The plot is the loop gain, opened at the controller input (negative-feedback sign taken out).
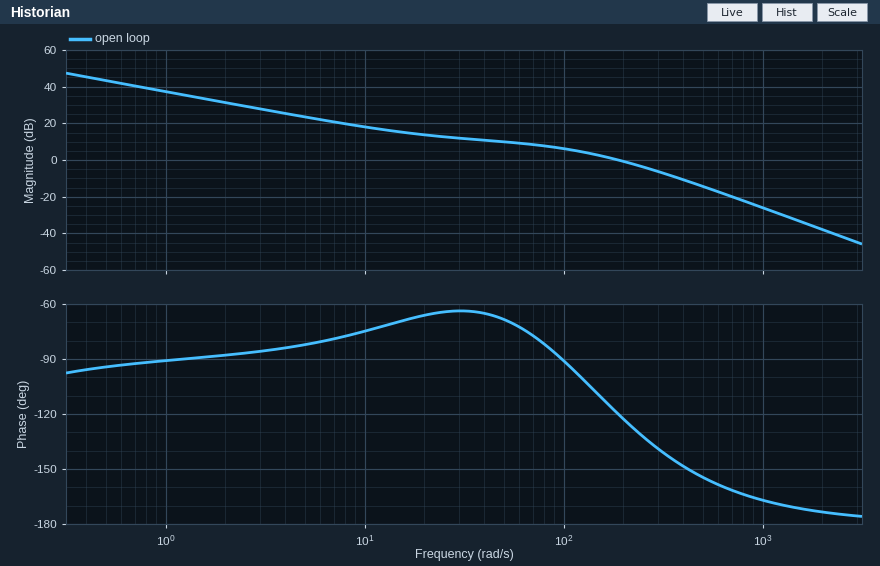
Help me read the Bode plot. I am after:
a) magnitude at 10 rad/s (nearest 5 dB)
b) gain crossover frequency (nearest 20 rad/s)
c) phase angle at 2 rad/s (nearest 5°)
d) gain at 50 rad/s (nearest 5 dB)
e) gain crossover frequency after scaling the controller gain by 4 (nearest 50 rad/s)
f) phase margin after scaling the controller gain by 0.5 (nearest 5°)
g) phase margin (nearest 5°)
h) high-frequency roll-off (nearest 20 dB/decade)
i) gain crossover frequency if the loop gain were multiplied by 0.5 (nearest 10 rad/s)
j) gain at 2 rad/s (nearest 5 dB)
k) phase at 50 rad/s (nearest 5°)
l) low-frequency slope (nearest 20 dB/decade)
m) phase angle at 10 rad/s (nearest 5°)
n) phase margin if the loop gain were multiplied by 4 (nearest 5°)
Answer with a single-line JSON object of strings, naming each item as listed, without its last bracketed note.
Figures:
{"magnitude at 10 rad/s": "20 dB", "gain crossover frequency": "180 rad/s", "phase angle at 2 rad/s": "-90°", "gain at 50 rad/s": "10 dB", "gain crossover frequency after scaling the controller gain by 4": "450 rad/s", "phase margin after scaling the controller gain by 0.5": "90°", "phase margin": "60°", "high-frequency roll-off": "-40 dB/decade", "gain crossover frequency if the loop gain were multiplied by 0.5": "100 rad/s", "gain at 2 rad/s": "30 dB", "phase at 50 rad/s": "-70°", "low-frequency slope": "-20 dB/decade", "phase angle at 10 rad/s": "-75°", "phase margin if the loop gain were multiplied by 4": "30°"}
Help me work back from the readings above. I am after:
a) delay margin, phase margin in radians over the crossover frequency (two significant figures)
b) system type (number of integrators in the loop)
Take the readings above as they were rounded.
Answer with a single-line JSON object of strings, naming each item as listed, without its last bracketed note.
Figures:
{"delay margin, phase margin in radians over the crossover frequency": "0.0058 s", "system type": "1"}
